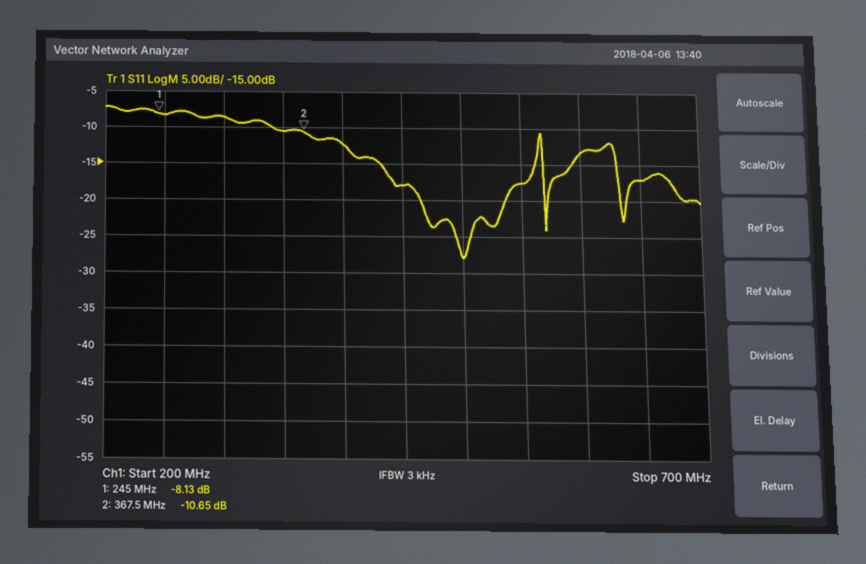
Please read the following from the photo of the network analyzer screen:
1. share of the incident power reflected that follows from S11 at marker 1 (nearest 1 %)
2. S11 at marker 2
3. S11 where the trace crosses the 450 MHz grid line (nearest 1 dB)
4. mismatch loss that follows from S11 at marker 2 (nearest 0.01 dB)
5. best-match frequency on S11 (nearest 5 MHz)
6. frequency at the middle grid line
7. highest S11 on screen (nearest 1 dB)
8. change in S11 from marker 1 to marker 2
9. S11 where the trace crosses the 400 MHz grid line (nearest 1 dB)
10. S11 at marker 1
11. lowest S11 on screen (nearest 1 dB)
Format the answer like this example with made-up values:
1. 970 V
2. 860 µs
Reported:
1. 15 %
2. -10.65 dB
3. -18 dB
4. 0.39 dB
5. 500 MHz
6. 450 MHz
7. -7 dB
8. -2.52 dB
9. -12 dB
10. -8.13 dB
11. -28 dB
